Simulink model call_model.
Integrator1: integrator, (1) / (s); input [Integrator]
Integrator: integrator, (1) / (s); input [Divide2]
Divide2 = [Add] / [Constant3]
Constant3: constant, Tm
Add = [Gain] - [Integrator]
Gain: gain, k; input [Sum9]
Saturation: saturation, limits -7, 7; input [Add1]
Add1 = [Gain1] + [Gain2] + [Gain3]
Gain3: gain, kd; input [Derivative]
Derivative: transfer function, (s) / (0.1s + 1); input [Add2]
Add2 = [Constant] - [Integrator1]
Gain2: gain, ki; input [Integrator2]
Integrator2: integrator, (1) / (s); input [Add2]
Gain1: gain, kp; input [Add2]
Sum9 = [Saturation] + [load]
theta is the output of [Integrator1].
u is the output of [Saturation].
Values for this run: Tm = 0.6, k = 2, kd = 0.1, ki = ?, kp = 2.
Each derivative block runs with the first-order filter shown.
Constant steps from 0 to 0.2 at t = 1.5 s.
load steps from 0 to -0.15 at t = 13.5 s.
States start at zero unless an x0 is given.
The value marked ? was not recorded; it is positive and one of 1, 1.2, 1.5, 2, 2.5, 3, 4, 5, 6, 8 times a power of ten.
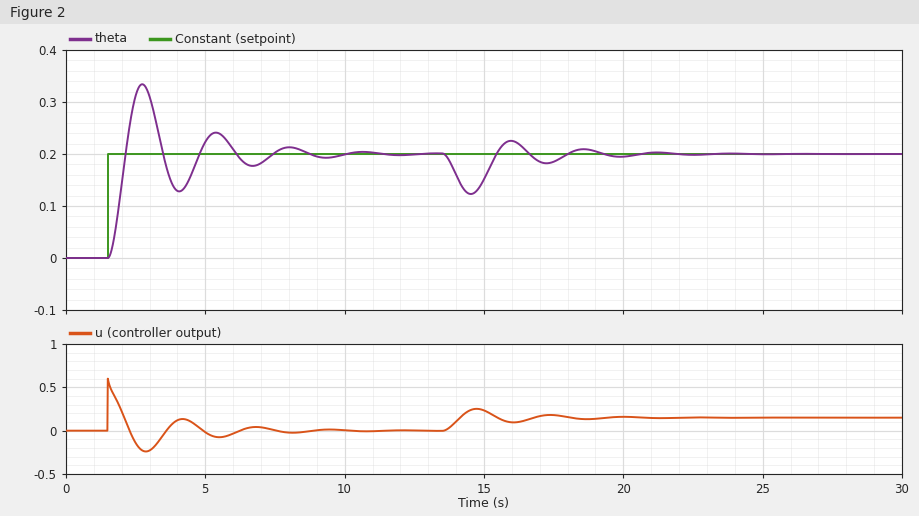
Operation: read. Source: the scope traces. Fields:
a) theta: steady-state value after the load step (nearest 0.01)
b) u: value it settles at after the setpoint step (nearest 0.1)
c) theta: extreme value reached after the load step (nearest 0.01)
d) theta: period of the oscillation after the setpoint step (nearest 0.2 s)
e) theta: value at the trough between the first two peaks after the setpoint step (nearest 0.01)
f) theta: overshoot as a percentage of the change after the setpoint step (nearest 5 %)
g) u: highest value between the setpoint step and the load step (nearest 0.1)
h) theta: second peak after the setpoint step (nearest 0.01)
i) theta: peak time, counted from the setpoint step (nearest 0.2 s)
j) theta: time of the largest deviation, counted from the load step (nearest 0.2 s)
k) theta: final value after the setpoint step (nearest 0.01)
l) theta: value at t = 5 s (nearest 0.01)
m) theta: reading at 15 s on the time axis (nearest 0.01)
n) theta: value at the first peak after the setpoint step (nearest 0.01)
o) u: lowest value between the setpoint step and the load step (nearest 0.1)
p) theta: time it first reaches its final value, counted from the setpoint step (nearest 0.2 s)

0.20
0.0
0.12
2.6 s
0.13
65 %
0.6
0.24
1.2 s
1.0 s
0.20
0.22
0.15
0.33
-0.2
0.6 s
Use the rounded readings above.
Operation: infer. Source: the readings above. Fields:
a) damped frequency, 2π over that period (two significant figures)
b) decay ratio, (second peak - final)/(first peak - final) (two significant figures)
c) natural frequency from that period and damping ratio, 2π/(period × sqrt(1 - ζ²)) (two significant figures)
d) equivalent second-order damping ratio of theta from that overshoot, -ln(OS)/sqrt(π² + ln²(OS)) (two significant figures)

2.4 rad/s
0.31
2.4 rad/s
0.14
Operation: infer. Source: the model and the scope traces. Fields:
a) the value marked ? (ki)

2
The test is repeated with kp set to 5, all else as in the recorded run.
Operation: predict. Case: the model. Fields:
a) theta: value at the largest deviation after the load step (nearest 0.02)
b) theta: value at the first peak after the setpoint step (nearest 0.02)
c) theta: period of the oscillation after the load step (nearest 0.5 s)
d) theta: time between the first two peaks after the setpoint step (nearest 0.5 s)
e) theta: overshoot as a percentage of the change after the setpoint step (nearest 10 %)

0.16
0.32
1.5 s
1.5 s
60 %
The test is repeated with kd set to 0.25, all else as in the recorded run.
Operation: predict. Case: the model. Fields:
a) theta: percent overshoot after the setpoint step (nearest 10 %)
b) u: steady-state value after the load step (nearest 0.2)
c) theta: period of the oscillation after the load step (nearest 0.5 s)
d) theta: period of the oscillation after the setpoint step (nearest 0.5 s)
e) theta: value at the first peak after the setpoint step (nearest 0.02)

50 %
0.2
3.0 s
3.0 s
0.30
